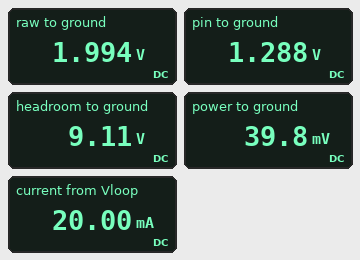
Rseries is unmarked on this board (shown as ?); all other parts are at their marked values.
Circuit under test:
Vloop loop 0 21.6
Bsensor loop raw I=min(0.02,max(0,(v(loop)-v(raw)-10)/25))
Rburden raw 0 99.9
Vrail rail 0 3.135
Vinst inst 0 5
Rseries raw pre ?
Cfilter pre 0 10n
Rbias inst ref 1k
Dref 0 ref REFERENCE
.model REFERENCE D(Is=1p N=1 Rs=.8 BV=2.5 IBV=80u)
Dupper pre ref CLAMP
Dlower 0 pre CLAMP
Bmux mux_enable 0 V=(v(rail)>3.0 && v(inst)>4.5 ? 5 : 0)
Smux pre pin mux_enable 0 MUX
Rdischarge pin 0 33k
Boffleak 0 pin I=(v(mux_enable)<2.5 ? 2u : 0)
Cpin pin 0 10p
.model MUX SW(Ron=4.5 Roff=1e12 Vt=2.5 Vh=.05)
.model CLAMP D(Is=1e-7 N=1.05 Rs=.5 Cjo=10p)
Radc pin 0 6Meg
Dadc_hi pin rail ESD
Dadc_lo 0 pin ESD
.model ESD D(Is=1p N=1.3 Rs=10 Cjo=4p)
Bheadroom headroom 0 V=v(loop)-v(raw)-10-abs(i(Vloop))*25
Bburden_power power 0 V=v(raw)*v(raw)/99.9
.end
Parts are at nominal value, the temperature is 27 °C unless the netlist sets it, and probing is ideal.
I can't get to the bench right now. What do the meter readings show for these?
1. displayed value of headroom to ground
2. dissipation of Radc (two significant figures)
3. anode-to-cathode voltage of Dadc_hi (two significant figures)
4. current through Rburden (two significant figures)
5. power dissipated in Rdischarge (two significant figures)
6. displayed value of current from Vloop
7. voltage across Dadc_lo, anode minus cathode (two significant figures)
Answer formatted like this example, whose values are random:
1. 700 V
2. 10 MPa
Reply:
1. 9.11 V
2. 280 nW
3. -1.8 V
4. 20 mA
5. 50 µW
6. 20.00 mA
7. -1.3 V
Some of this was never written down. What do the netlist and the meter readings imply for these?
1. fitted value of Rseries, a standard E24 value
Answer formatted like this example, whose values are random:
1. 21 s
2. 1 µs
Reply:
1. 18 kΩ
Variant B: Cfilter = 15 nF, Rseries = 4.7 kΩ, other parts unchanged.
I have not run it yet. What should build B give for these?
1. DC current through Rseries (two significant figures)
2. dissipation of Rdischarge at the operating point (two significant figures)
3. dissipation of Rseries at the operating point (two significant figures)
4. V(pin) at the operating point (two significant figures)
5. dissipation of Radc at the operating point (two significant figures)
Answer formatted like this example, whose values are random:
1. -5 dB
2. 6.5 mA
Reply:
1. 53 µA
2. 92 µW
3. 13 µW
4. 1.7 V
5. 510 nW
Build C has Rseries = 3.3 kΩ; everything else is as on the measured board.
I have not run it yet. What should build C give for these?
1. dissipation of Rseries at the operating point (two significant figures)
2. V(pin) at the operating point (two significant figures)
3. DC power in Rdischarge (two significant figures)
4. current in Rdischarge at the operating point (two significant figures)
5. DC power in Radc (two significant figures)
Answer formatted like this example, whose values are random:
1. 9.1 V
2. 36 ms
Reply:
1. 10 µW
2. 1.8 V
3. 99 µW
4. 55 µA
5. 550 nW
